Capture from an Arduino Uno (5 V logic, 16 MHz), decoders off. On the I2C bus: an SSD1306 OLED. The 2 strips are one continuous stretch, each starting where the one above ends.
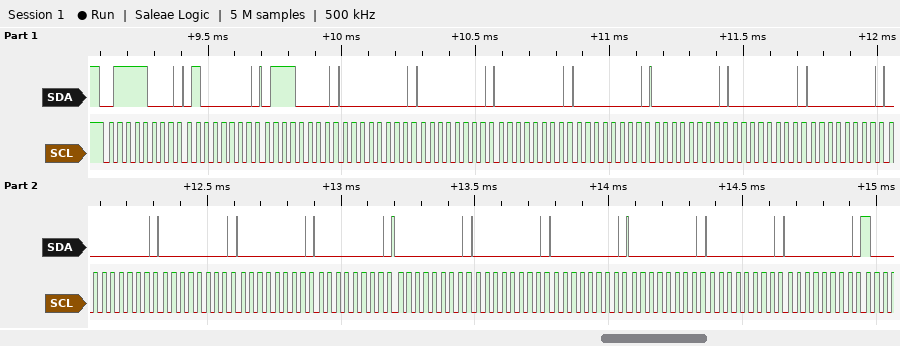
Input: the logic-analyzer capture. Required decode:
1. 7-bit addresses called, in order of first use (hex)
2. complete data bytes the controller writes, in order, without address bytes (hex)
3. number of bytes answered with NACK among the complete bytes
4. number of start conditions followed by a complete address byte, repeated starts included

0x3C
40 70 00 00 00 00 00 00 00 00 00 00 00 00 00 00 00 00 00
0
1
